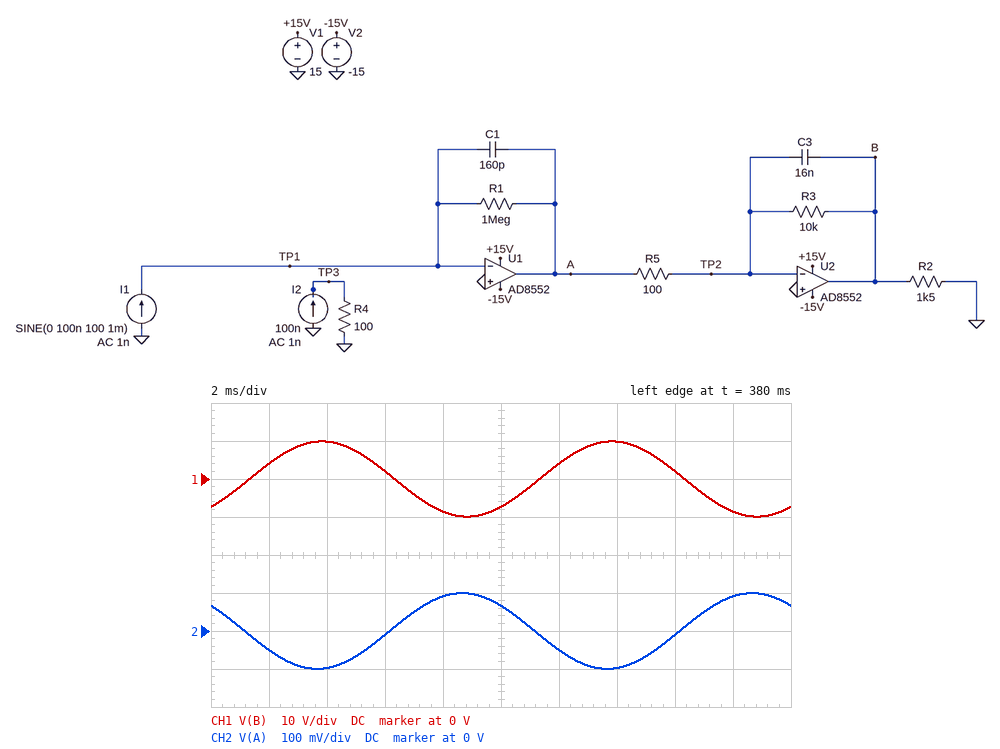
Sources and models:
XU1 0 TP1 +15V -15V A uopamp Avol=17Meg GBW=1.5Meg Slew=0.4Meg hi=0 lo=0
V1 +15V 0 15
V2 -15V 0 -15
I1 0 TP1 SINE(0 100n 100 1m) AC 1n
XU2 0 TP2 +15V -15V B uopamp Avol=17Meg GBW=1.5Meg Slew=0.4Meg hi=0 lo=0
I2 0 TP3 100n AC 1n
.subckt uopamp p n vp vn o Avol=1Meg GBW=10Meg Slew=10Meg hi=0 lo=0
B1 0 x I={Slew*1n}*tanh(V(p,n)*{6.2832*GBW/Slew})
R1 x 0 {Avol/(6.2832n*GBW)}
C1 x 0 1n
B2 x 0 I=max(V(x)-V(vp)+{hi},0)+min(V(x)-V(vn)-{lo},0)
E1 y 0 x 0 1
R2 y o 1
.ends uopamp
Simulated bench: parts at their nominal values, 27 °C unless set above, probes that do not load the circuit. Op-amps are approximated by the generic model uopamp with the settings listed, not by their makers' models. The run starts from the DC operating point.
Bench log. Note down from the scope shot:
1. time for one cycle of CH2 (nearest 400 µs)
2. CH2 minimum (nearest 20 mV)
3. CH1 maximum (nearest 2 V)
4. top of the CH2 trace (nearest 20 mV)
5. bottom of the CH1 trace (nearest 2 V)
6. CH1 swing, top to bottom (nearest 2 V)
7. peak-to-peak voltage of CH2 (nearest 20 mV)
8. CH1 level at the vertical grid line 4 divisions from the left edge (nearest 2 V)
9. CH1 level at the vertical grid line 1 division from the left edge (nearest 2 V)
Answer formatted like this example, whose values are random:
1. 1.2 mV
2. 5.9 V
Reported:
1. 10.0 ms
2. -100 mV
3. 10 V
4. 100 mV
5. -10 V
6. 20 V
7. 200 mV
8. -8 V
9. 4 V
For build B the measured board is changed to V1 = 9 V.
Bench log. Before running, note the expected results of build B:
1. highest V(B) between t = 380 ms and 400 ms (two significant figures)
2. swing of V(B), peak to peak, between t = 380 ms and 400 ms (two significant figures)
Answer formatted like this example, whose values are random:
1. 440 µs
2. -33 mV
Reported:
1. 9.0 V
2. 19 V
